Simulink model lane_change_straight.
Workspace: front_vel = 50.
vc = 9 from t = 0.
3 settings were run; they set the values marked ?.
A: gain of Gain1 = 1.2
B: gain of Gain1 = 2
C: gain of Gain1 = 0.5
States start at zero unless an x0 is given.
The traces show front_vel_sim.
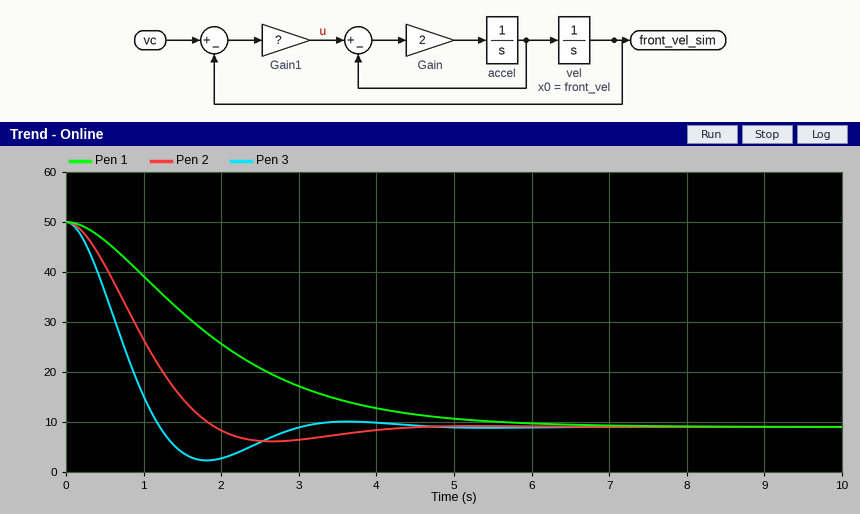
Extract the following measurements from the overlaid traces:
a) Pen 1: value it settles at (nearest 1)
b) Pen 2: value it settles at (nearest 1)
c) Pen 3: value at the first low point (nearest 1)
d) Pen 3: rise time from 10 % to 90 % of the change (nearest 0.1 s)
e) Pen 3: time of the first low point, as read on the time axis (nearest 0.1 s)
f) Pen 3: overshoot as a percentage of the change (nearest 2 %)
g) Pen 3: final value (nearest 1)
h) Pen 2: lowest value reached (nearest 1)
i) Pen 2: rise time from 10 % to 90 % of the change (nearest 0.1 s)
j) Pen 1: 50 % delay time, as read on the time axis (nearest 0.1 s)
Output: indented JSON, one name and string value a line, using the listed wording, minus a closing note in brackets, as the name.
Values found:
{
  "Pen 1: value it settles at": "9",
  "Pen 2: value it settles at": "9",
  "Pen 3: value at the first low point": "2",
  "Pen 3: rise time from 10 % to 90 % of the change": "0.8 s",
  "Pen 3: time of the first low point, as read on the time axis": "1.8 s",
  "Pen 3: overshoot as a percentage of the change": "16 %",
  "Pen 3: final value": "9",
  "Pen 2: lowest value reached": "6",
  "Pen 2: rise time from 10 % to 90 % of the change": "1.3 s",
  "Pen 1: 50 % delay time, as read on the time axis": "1.7 s"
}
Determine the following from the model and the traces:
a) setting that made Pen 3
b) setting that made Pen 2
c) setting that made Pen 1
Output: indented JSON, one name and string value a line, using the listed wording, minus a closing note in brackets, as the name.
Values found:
{
  "setting that made Pen 3": "B",
  "setting that made Pen 2": "A",
  "setting that made Pen 1": "C"
}
